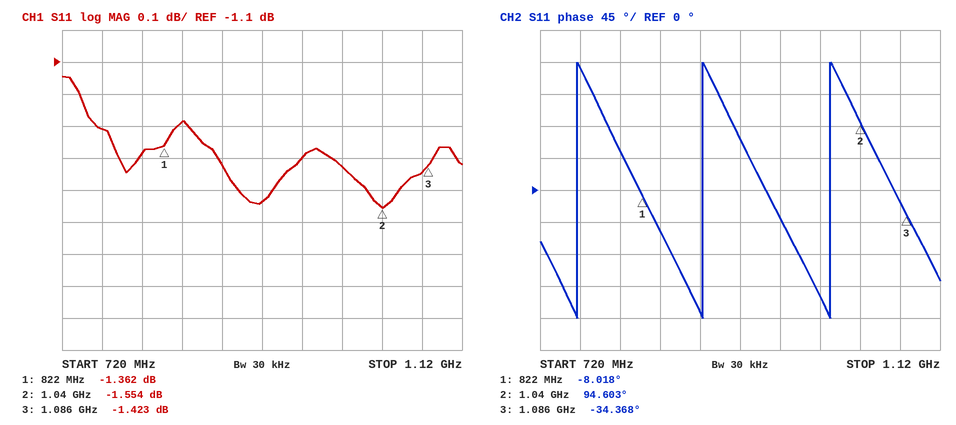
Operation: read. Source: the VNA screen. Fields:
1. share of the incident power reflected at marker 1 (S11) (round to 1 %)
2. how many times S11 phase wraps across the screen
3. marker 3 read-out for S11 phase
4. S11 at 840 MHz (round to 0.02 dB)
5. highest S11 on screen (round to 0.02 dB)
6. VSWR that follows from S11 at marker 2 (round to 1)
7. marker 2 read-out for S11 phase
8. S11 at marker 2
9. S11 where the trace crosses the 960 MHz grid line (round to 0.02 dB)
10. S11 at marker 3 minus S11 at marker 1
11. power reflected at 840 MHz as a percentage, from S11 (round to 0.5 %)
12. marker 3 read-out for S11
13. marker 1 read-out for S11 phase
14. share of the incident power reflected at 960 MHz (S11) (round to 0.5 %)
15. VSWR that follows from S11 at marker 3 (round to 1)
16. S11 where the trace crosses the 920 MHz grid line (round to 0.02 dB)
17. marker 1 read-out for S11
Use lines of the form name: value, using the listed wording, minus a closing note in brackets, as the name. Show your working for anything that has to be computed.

share of the incident power reflected at marker 1 (S11): 10^(-1.362/10) ≈ 73 %
how many times S11 phase wraps across the screen: 3
marker 3 read-out for S11 phase: -34.368°
S11 at 840 MHz: -1.28 dB
highest S11 on screen: -1.14 dB
VSWR that follows from S11 at marker 2: (1 + 0.8362)/(1 − 0.8362) ≈ 11
marker 2 read-out for S11 phase: 94.603°
S11 at marker 2: -1.554 dB
S11 where the trace crosses the 960 MHz grid line: -1.40 dB
S11 at marker 3 minus S11 at marker 1: -1.423 − (-1.362) = -0.061 dB
power reflected at 840 MHz as a percentage, from S11: 10^(-1.28/10) ≈ 74.5 %
marker 3 read-out for S11: -1.423 dB
marker 1 read-out for S11 phase: -8.018°
share of the incident power reflected at 960 MHz (S11): 10^(-1.4/10) ≈ 72.4 %, so 72.5 % to the nearest 0.5 %
VSWR that follows from S11 at marker 3: (1 + 0.8489)/(1 − 0.8489) ≈ 12
S11 where the trace crosses the 920 MHz grid line: -1.54 dB
marker 1 read-out for S11: -1.362 dB
